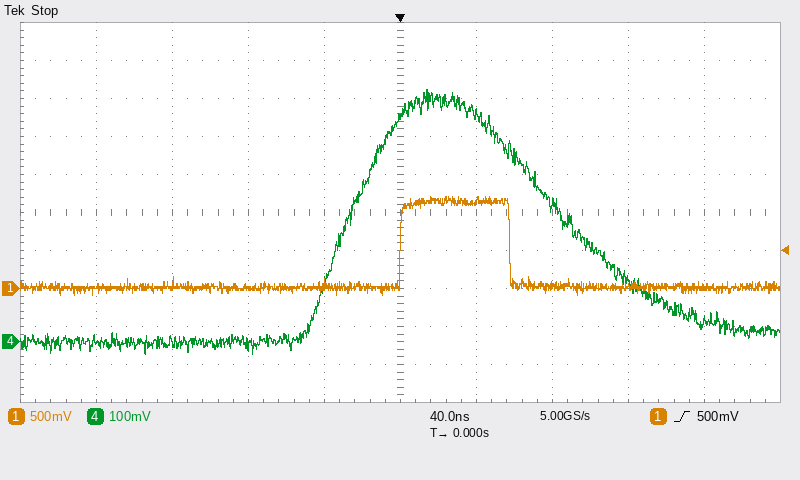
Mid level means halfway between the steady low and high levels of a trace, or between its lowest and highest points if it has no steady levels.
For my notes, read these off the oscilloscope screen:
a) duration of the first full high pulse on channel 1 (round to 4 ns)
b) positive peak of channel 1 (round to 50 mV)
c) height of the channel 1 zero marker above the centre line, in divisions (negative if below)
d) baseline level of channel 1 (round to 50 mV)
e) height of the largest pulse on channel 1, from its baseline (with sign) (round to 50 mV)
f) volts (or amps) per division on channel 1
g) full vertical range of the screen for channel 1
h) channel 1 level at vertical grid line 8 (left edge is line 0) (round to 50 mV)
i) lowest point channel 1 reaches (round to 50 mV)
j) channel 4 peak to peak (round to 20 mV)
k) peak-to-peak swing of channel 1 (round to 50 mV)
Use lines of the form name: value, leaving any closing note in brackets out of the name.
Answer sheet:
duration of the first full high pulse on channel 1: 56 ns
positive peak of channel 1: 1.20 V
height of the channel 1 zero marker above the centre line, in divisions: -2.0 div
baseline level of channel 1: 0 mV
height of the largest pulse on channel 1, from its baseline (with sign): +1.20 V
volts (or amps) per division on channel 1: 500 mV
full vertical range of the screen for channel 1: 5 V
channel 1 level at vertical grid line 8 (left edge is line 0): 0 mV
lowest point channel 1 reaches: -100 mV
channel 4 peak to peak: 700 mV
peak-to-peak swing of channel 1: 1.30 V
